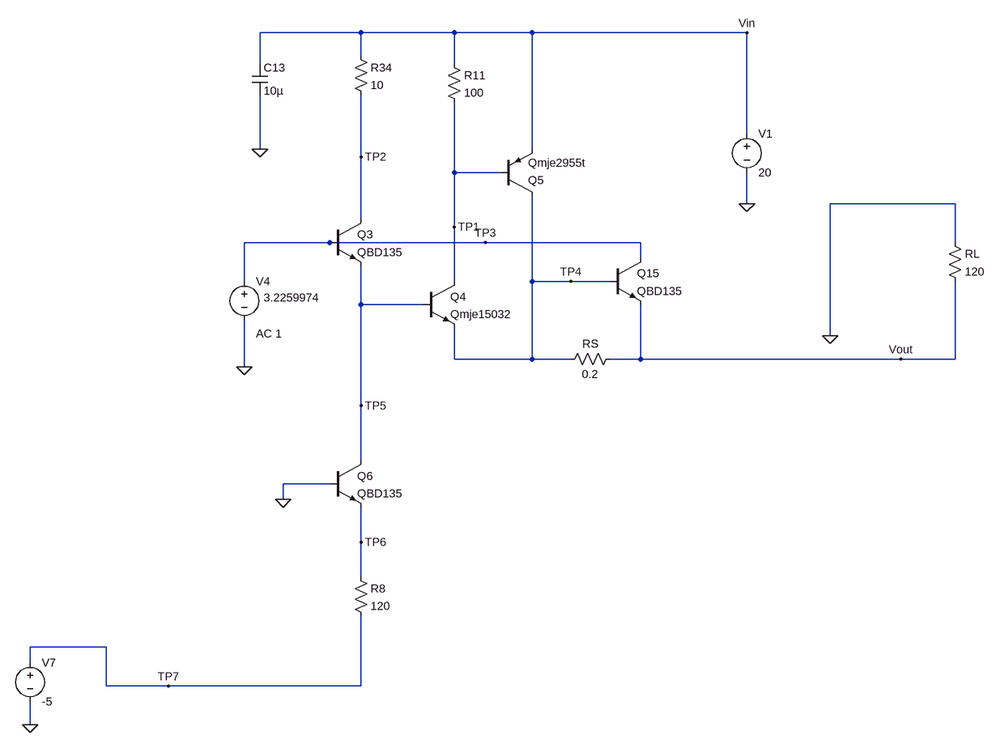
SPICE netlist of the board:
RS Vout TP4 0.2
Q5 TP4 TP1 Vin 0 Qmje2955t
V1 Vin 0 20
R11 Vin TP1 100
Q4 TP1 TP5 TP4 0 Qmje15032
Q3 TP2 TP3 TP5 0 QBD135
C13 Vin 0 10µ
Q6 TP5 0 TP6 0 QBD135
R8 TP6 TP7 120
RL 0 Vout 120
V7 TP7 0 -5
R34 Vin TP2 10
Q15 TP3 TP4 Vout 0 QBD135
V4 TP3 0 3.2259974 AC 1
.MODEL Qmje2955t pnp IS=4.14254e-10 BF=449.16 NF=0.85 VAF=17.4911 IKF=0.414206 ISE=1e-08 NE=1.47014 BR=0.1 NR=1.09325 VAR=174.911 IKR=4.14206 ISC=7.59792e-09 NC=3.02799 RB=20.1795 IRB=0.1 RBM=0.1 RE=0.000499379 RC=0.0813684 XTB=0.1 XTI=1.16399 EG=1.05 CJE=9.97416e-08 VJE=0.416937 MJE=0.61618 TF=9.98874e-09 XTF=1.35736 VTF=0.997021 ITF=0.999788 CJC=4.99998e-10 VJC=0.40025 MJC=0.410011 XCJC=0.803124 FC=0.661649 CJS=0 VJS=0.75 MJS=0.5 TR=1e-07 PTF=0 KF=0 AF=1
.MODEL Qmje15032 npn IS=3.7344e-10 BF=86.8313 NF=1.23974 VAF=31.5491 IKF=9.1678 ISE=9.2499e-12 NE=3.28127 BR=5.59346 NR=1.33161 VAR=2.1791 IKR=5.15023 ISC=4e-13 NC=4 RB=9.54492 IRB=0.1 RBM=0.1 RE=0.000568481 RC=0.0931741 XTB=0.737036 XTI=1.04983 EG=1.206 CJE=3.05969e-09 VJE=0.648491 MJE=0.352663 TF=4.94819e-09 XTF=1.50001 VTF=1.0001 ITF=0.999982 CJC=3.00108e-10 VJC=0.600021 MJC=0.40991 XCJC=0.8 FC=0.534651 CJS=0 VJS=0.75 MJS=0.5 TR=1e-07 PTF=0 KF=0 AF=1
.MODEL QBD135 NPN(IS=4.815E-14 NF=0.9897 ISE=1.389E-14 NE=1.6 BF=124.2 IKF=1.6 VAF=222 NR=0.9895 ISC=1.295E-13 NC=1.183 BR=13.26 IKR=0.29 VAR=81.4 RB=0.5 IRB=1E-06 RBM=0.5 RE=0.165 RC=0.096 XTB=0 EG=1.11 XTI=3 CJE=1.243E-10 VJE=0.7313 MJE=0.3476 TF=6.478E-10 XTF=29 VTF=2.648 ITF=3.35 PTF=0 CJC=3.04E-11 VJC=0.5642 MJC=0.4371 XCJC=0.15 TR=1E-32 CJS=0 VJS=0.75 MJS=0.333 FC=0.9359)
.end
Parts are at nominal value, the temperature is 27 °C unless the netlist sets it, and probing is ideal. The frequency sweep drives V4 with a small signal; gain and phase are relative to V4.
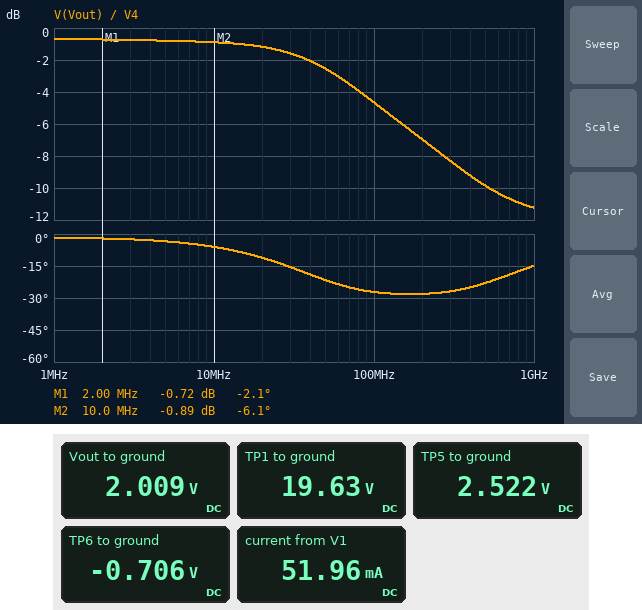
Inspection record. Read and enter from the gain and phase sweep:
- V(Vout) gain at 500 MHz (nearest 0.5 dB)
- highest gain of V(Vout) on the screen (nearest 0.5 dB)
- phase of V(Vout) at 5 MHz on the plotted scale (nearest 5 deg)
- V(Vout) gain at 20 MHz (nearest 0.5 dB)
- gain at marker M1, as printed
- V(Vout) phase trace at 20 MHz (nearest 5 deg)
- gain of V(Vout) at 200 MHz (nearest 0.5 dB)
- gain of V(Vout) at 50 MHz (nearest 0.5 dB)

-10.0 dB
-0.5 dB
-5 deg
-1.0 dB
-0.72 dB
-10 deg
-7.0 dB
-2.5 dB
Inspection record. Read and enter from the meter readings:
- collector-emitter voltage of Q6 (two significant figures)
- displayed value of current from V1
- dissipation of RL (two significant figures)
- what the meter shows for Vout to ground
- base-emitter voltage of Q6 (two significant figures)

3.2 V
51.96 mA
34 mW
2.009 V
710 mV
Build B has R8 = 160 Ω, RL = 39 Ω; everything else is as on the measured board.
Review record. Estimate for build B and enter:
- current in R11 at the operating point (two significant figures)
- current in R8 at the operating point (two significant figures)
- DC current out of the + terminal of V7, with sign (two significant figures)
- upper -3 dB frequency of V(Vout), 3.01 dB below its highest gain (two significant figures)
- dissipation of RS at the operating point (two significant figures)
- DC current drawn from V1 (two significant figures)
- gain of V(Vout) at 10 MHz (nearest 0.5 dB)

4.0 mA
27 mA
-27 mA
32 MHz
530 µW
78 mA
-2.5 dB
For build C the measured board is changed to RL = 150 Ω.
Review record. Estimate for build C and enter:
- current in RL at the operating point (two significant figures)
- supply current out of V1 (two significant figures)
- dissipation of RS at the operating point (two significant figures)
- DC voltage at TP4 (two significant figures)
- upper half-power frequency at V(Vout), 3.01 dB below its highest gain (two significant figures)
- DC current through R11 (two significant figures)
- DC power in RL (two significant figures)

13 mA
49 mA
36 µW
2.0 V
62 MHz
3.6 mA
27 mW
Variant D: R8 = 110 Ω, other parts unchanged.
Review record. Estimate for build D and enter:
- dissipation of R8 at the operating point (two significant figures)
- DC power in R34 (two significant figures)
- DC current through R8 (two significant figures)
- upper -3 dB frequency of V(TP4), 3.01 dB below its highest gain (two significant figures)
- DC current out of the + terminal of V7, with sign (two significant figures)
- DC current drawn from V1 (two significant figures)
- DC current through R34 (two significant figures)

170 mW
15 mW
39 mA
61 MHz
-39 mA
55 mA
38 mA
